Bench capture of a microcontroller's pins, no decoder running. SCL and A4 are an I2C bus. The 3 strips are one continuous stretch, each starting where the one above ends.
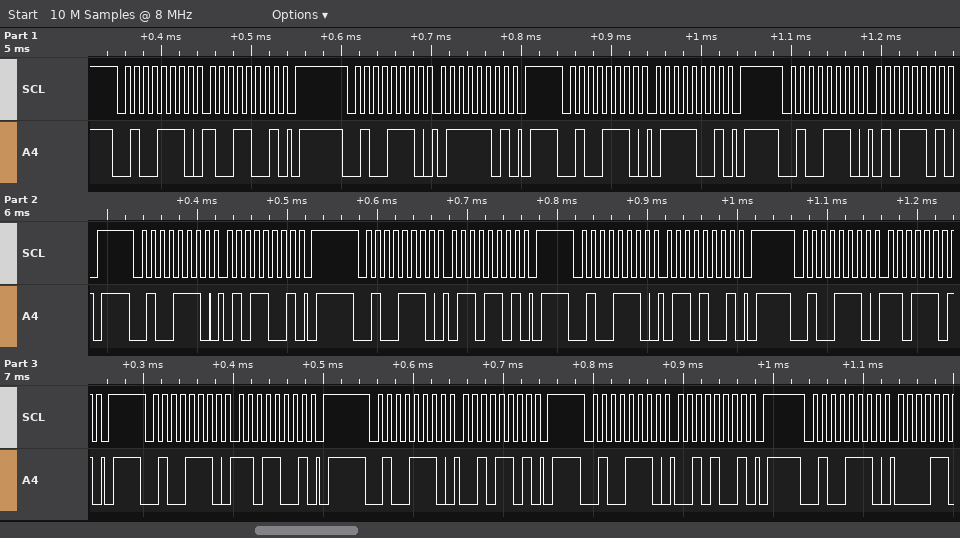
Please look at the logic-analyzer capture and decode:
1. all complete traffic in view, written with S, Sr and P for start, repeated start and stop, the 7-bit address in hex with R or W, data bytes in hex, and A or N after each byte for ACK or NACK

S 27W A 99 A P S 27W A 7D A P S 27W A 79 A P S 27W A 5D A P S 27W A 59 A P S 27W A 6D A P S 27W A 69 A P S 27W A DD A P S 27W A D9 A P S 27W A 2D A P S 27W A 29 A P S 27W A
